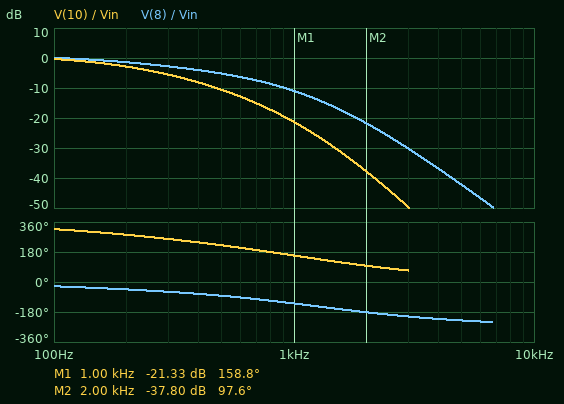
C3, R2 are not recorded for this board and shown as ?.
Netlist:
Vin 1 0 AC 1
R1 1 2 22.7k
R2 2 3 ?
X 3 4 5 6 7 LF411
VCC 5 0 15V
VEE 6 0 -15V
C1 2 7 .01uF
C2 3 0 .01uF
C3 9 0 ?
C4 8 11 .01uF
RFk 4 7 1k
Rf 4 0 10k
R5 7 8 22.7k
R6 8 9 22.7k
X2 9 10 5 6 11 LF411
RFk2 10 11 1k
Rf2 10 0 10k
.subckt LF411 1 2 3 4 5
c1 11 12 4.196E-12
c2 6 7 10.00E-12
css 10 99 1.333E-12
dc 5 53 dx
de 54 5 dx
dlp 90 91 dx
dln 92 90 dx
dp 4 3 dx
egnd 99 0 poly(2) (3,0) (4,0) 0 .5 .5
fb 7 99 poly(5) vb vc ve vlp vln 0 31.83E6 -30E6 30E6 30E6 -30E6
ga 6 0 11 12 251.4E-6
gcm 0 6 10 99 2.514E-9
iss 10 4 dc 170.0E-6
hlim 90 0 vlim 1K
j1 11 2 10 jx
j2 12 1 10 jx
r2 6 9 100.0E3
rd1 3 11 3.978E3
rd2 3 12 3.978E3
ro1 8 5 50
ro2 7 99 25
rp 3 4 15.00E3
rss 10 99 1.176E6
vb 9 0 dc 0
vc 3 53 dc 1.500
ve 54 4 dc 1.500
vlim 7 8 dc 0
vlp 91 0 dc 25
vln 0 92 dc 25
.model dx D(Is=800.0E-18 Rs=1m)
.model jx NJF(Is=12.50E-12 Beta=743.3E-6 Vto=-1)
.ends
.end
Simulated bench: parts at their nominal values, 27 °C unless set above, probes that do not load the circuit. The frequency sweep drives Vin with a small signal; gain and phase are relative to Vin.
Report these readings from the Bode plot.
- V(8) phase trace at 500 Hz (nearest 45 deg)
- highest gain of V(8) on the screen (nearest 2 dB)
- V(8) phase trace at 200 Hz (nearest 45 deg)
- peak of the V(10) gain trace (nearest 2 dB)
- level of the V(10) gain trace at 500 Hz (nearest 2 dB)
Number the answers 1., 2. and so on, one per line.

1. -90 deg
2. 0 dB
3. -45 deg
4. 0 dB
5. -10 dB
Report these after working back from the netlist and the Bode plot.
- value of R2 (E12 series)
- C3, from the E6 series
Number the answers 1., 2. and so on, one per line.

1. 8.2 kΩ
2. 22 nF
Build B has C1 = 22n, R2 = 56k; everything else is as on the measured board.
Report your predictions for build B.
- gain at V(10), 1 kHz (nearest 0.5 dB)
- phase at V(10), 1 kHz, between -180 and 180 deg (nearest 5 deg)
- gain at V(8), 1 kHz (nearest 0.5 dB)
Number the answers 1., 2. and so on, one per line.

1. -37.0 dB
2. 85 deg
3. -26.5 dB
